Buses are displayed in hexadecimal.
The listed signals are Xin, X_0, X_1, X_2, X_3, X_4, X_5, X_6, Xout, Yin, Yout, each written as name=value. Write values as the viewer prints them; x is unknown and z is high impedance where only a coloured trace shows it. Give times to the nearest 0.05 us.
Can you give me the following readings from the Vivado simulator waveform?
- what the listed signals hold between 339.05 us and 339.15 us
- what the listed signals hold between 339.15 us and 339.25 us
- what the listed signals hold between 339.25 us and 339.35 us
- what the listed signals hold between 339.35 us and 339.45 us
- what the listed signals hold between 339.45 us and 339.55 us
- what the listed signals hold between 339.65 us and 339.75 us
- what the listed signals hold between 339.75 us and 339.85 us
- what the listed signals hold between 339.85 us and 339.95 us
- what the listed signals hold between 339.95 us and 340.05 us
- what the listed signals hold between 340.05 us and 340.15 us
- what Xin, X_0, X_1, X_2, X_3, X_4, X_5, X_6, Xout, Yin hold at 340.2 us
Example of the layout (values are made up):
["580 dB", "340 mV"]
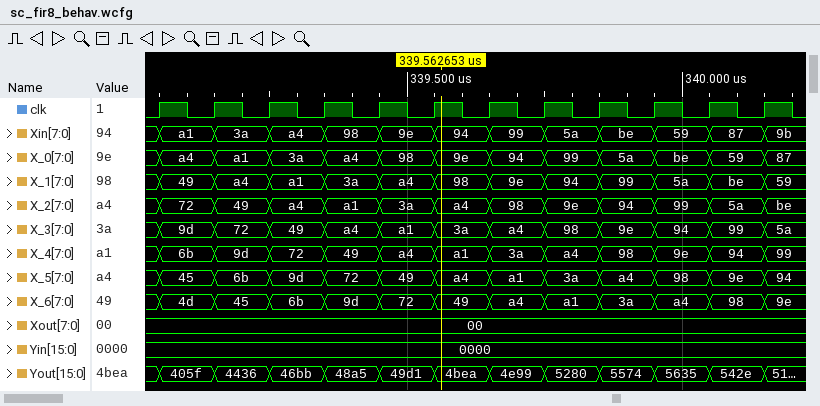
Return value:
["Xin=a1, X_0=a4, X_1=49, X_2=72, X_3=9d, X_4=6b, X_5=45, X_6=4d, Xout=00, Yin=0000, Yout=405f", "Xin=3a, X_0=a1, X_1=a4, X_2=49, X_3=72, X_4=9d, X_5=6b, X_6=45, Xout=00, Yin=0000, Yout=4436", "Xin=a4, X_0=3a, X_1=a1, X_2=a4, X_3=49, X_4=72, X_5=9d, X_6=6b, Xout=00, Yin=0000, Yout=46bb", "Xin=98, X_0=a4, X_1=3a, X_2=a1, X_3=a4, X_4=49, X_5=72, X_6=9d, Xout=00, Yin=0000, Yout=48a5", "Xin=9e, X_0=98, X_1=a4, X_2=3a, X_3=a1, X_4=a4, X_5=49, X_6=72, Xout=00, Yin=0000, Yout=49d1", "Xin=99, X_0=94, X_1=9e, X_2=98, X_3=a4, X_4=3a, X_5=a1, X_6=a4, Xout=00, Yin=0000, Yout=4e99", "Xin=5a, X_0=99, X_1=94, X_2=9e, X_3=98, X_4=a4, X_5=3a, X_6=a1, Xout=00, Yin=0000, Yout=5280", "Xin=be, X_0=5a, X_1=99, X_2=94, X_3=9e, X_4=98, X_5=a4, X_6=3a, Xout=00, Yin=0000, Yout=5574", "Xin=59, X_0=be, X_1=5a, X_2=99, X_3=94, X_4=9e, X_5=98, X_6=a4, Xout=00, Yin=0000, Yout=5635", "Xin=87, X_0=59, X_1=be, X_2=5a, X_3=99, X_4=94, X_5=9e, X_6=98, Xout=00, Yin=0000, Yout=542e", "Xin=9b, X_0=87, X_1=59, X_2=be, X_3=5a, X_4=99, X_5=94, X_6=9e, Xout=00, Yin=0000"]
